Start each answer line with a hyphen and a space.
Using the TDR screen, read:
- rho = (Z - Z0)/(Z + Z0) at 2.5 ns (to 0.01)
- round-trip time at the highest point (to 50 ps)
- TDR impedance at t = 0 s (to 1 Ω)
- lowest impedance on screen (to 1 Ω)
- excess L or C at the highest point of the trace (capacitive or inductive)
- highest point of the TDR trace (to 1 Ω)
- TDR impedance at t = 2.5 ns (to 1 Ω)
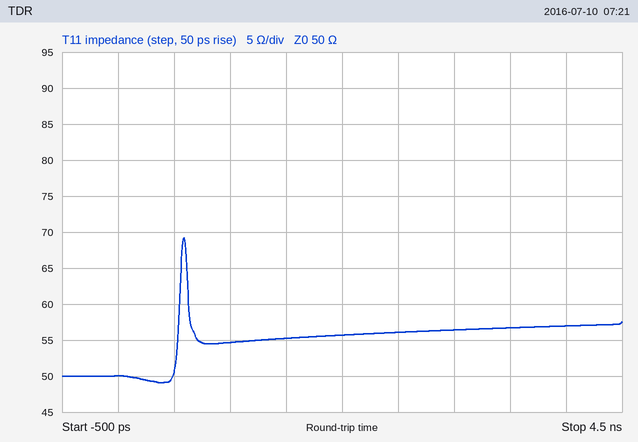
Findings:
- +0.06
- 600 ps
- 50 Ω
- 49 Ω
- inductive
- 69 Ω
- 56 Ω
